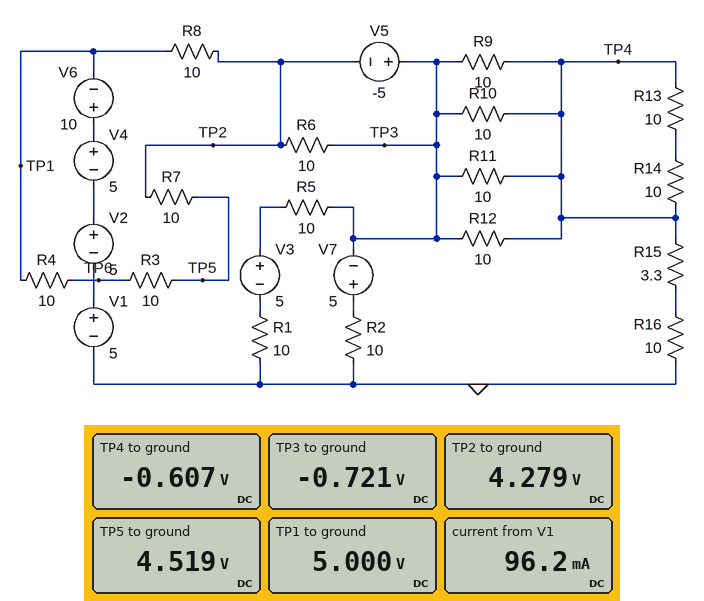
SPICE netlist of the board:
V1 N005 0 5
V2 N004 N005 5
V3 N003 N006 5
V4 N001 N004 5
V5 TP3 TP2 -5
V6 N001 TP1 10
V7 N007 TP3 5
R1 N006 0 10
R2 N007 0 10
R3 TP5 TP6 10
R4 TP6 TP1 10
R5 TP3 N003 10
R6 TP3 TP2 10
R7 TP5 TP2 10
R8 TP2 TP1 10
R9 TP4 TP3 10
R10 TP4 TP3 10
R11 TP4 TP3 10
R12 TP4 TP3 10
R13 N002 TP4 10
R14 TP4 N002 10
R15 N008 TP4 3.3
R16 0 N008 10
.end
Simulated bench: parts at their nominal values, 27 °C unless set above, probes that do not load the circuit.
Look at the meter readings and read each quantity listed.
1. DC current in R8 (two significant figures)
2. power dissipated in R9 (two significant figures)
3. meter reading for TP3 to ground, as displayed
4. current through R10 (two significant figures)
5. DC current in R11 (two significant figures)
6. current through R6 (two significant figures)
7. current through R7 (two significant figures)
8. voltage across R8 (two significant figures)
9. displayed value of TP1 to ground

72 mA
1.3 mW
-0.721 V
11 mA
11 mA
500 mA
24 mA
720 mV
5.000 V
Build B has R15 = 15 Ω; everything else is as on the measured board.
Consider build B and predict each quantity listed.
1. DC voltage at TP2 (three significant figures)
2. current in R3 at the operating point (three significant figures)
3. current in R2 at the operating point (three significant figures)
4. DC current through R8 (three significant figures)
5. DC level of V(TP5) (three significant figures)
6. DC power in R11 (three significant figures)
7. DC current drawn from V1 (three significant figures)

4.22 V
26.1 mA
422 mA
78.2 mA
4.48 V
505 µW
104 mA
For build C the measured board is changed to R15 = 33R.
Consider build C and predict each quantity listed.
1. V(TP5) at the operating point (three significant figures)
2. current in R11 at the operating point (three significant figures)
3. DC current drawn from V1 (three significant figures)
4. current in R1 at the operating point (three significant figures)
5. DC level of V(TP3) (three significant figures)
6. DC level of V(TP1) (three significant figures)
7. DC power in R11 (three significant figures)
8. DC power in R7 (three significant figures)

4.45 V
4.50 mA
109 mA
291 mA
-819 mV
5.00 V
202 µW
7.45 mW
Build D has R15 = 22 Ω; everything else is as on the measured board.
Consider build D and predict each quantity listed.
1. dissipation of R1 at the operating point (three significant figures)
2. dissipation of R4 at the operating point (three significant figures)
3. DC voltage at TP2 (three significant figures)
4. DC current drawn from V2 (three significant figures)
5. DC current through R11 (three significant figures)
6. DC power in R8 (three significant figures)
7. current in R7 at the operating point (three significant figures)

841 mW
7.12 mW
4.20 V
107 mA
5.80 mA
64.1 mW
26.7 mA
